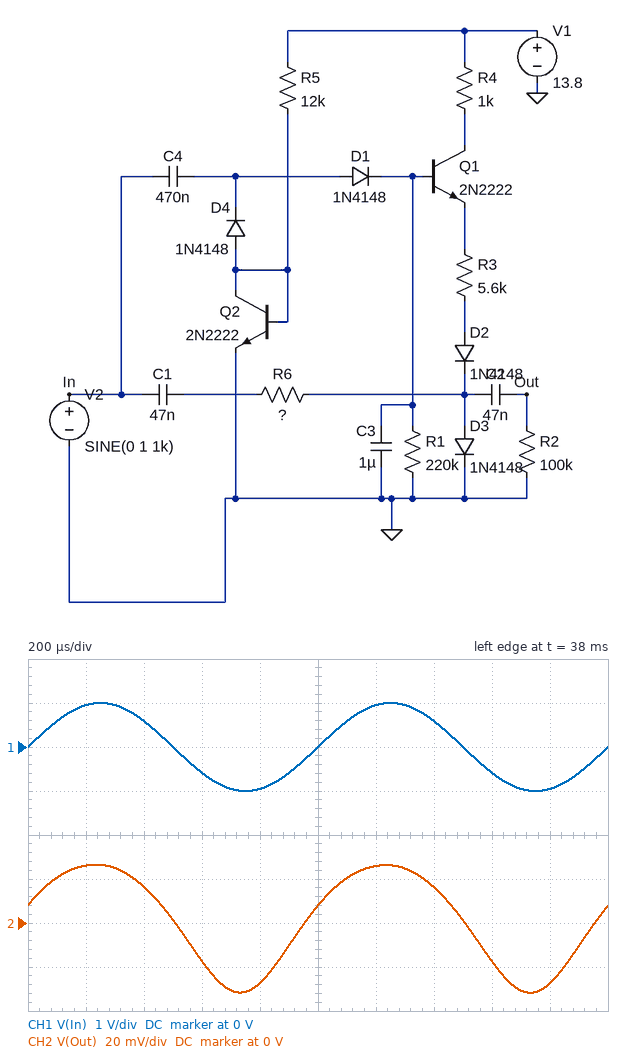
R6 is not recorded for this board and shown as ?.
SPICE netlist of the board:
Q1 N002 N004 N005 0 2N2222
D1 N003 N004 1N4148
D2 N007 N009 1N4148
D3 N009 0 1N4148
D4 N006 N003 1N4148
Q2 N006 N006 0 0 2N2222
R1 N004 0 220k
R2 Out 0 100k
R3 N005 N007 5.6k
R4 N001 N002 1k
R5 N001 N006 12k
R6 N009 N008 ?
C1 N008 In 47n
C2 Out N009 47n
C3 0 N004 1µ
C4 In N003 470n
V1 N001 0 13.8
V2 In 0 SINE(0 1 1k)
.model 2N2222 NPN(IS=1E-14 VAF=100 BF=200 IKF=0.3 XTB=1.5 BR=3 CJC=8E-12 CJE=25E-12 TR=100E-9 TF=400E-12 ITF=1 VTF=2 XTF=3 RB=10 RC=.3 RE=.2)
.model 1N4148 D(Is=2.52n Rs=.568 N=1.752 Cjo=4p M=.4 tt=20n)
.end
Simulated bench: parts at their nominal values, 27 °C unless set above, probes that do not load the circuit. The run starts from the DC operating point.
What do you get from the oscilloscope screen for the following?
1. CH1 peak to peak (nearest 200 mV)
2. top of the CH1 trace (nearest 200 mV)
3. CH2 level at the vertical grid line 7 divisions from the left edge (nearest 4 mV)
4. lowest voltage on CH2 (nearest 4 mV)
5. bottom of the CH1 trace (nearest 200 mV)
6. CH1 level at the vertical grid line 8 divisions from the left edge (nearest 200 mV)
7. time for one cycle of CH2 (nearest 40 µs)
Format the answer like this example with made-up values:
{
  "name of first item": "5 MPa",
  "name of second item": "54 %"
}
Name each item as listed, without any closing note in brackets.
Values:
{
  "CH1 peak to peak": "2.0 V",
  "top of the CH1 trace": "1.0 V",
  "CH2 level at the vertical grid line 7 divisions from the left edge": "16 mV",
  "lowest voltage on CH2": "-32 mV",
  "bottom of the CH1 trace": "-1.0 V",
  "CH1 level at the vertical grid line 8 divisions from the left edge": "-600 mV",
  "time for one cycle of CH2": "1.00 ms"
}
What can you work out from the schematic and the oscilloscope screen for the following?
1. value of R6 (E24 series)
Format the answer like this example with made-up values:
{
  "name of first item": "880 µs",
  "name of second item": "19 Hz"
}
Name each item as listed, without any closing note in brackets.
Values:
{
  "value of R6": "33 kΩ"
}
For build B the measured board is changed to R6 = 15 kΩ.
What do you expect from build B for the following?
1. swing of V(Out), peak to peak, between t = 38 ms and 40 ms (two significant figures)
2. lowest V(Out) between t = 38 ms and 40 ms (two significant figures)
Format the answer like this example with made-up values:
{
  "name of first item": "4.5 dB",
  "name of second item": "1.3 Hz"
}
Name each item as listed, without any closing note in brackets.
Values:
{
  "swing of V(Out), peak to peak, between t = 38 ms and 40 ms": "160 mV",
  "lowest V(Out) between t = 38 ms and 40 ms": "-100 mV"
}
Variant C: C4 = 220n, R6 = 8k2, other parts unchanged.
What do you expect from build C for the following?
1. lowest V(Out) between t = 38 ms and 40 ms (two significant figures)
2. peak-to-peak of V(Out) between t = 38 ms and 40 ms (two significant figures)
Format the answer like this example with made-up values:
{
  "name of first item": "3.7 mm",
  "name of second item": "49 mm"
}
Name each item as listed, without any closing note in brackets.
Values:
{
  "lowest V(Out) between t = 38 ms and 40 ms": "-220 mV",
  "peak-to-peak of V(Out) between t = 38 ms and 40 ms": "350 mV"
}
